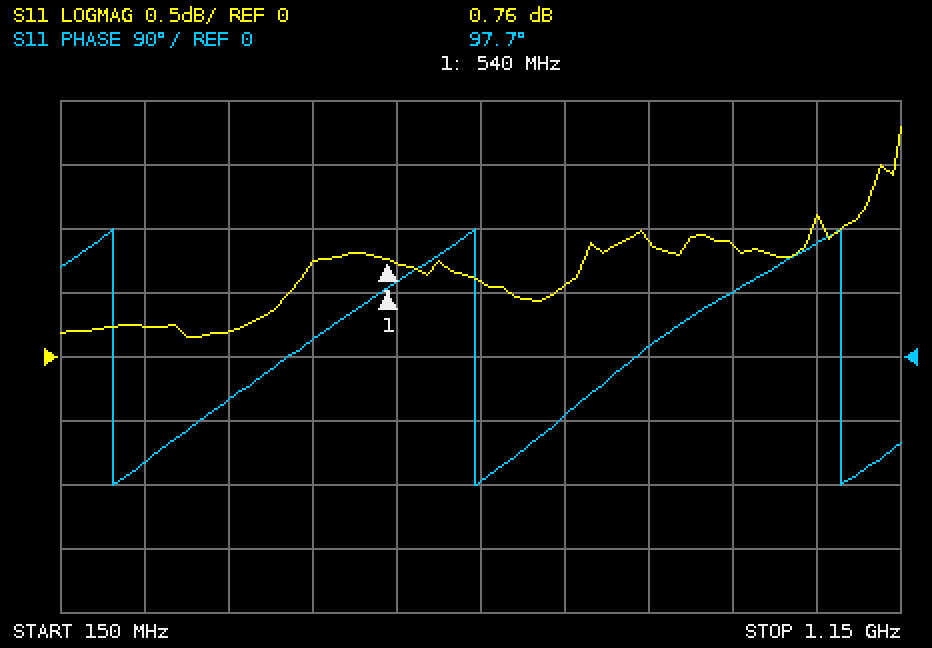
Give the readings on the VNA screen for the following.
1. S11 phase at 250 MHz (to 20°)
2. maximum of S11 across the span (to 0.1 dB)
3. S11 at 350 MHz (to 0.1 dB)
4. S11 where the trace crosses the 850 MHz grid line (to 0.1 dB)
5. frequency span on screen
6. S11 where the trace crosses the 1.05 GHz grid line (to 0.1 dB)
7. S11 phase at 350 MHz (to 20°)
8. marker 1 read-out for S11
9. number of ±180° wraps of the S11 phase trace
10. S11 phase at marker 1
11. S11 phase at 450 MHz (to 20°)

-140°
1.8 dB
0.2 dB
0.9 dB
1 GHz
1.1 dB
-60°
0.76 dB
3
97.7°
20°
